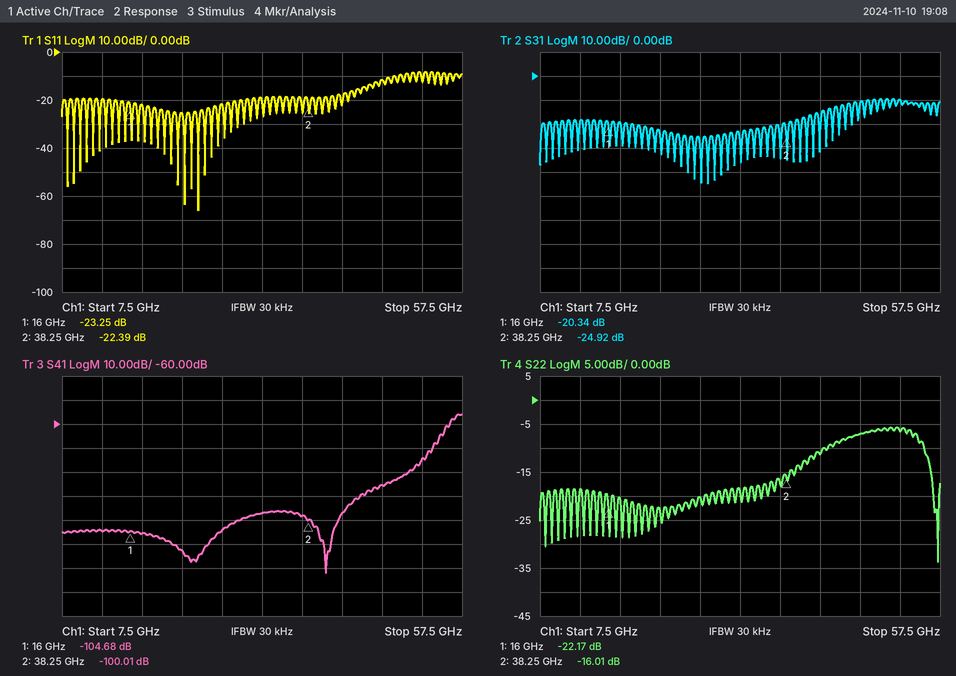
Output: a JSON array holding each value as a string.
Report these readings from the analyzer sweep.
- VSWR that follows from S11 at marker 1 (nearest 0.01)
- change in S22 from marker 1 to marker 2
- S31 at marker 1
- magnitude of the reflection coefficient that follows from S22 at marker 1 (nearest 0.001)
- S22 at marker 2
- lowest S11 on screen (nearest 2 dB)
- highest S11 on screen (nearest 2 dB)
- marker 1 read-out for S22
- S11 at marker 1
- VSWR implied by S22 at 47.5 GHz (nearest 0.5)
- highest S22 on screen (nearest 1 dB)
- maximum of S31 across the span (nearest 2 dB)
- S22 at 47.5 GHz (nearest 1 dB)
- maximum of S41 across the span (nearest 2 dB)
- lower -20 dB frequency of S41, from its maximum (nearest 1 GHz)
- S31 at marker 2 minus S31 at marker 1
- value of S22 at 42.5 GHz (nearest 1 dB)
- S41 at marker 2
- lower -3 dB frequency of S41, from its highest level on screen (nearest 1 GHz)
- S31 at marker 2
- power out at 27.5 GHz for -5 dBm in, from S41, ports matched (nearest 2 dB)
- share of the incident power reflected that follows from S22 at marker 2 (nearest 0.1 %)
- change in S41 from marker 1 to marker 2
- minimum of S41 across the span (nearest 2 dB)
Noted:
["1.15", "6.16 dB", "-20.34 dB", "0.078", "-16.01 dB", "-66 dB", "-8 dB", "-22.17 dB", "-23.25 dB", "2.5", "-6 dB", "-10 dB", "-7 dB", "-56 dB", "52 GHz", "-4.58 dB", "-11 dB", "-100.01 dB", "56 GHz", "-24.92 dB", "-110 dBm", "2.5 %", "4.67 dB", "-122 dB"]
